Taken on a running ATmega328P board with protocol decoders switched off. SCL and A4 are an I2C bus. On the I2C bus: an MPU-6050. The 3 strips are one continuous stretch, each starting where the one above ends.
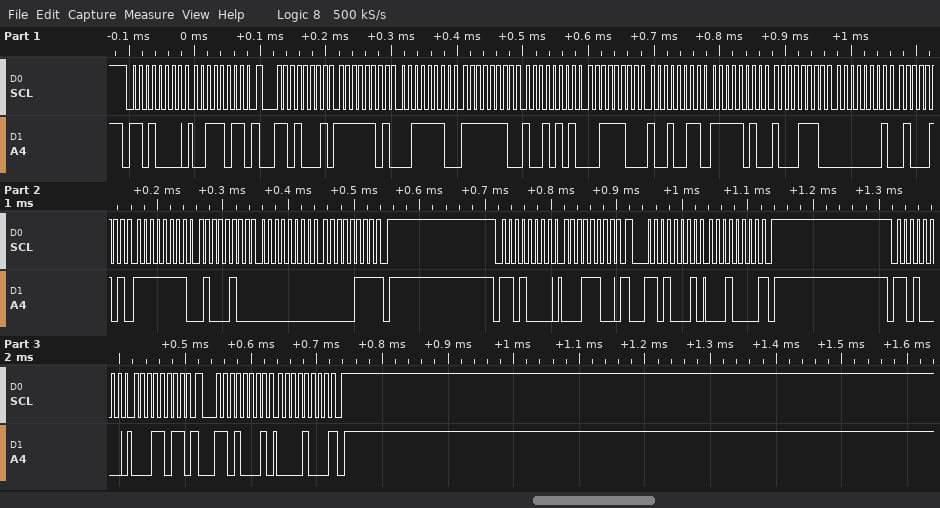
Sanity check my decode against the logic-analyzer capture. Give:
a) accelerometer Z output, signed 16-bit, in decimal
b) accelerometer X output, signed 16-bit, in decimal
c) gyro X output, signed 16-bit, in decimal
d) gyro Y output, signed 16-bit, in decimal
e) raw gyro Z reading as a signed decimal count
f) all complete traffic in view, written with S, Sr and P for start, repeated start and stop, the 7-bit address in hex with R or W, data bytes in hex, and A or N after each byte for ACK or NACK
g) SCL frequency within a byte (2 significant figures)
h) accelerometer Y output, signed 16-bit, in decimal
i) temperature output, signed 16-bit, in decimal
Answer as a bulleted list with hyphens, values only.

- 15507
- -706
- 325
- -188
- 7
- S 68W A 3B A Sr 68R A FD A 3E A FE A 95 A 3C A 93 A FA A 8E A 01 A 45 A FF A 44 A 00 A 07 N P S 68W A 1C A Sr 68R A 10 N P S 68W A 1B A Sr 68R A 08 N P
- 100 kHz
- -363
- -1394
